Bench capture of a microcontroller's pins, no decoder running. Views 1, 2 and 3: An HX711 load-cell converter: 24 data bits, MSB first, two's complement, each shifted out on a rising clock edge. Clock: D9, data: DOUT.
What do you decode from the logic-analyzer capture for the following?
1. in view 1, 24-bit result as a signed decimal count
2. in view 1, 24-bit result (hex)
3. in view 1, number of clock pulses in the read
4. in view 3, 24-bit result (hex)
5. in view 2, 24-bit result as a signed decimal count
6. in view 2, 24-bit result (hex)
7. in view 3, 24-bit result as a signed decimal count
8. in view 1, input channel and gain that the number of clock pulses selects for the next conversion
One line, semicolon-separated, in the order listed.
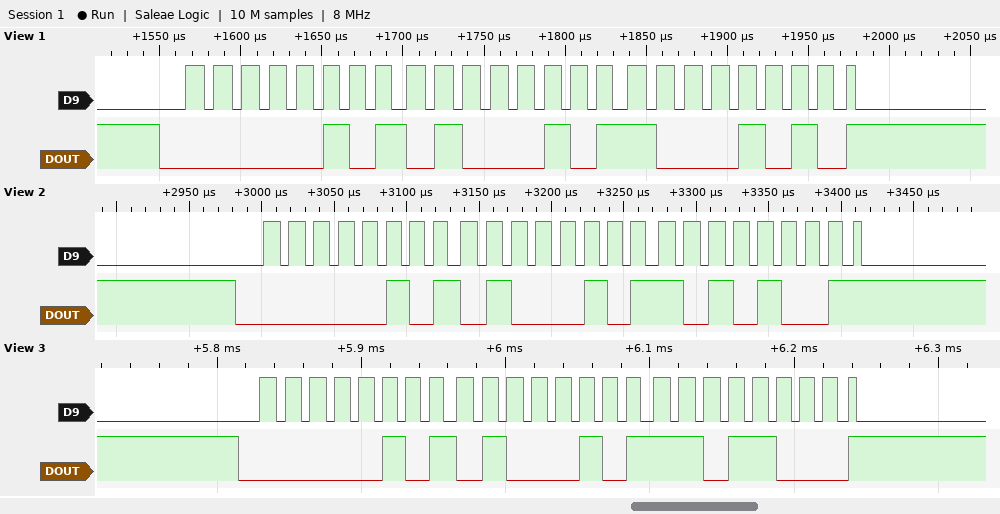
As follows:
345482; 0x05458A; 25; 0x0545D8; 345513; 0x0545A9; 345560; channel A, gain 128
